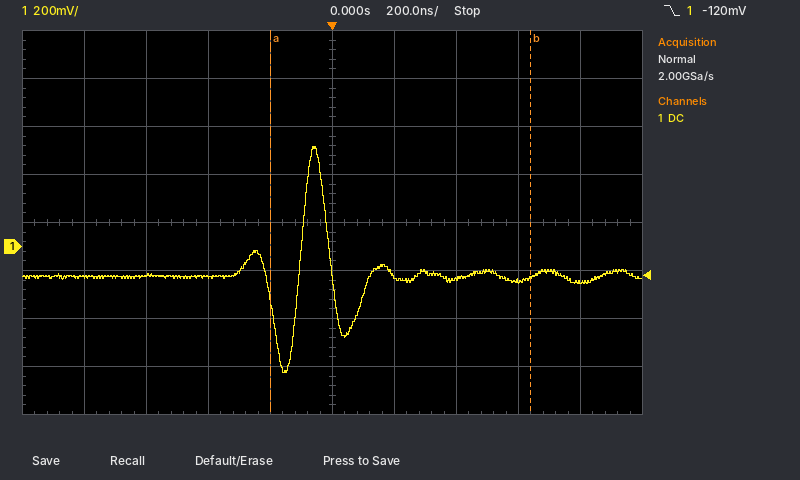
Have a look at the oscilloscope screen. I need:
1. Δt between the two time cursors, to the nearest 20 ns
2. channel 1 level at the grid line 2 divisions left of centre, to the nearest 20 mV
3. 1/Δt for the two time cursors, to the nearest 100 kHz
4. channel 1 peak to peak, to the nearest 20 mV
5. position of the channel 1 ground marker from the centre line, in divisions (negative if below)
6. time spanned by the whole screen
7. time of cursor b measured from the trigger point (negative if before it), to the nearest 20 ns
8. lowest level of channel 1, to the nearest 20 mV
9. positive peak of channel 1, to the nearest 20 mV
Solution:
840 ns
-120 mV
1.2 MHz
940 mV
-0.5 div
2 µs
+640 ns
-520 mV
420 mV
